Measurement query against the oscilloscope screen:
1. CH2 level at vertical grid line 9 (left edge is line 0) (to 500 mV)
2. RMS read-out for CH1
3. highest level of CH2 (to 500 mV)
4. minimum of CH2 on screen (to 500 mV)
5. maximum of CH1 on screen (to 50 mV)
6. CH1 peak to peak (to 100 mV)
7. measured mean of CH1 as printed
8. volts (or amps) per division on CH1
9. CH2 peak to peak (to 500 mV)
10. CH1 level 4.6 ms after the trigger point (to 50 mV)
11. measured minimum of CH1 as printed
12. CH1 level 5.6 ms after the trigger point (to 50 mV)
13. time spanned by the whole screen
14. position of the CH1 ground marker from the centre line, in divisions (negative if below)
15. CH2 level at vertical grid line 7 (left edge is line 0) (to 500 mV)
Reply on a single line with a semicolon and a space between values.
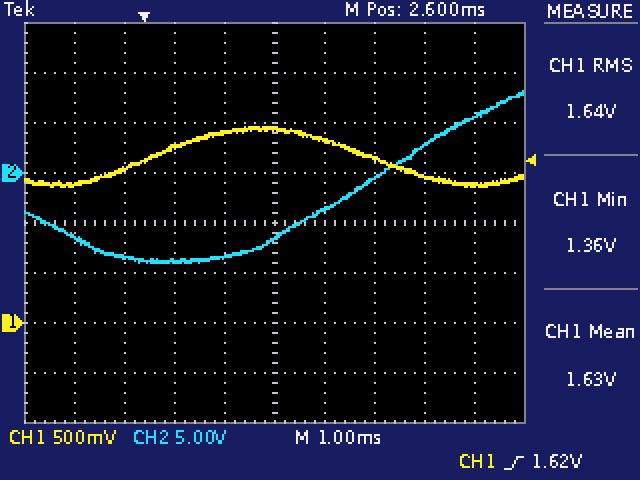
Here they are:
5.5 V; 1.64 V; 8.0 V; -9.0 V; 1.95 V; 600 mV; 1.63 V; 500 mV; 17.0 V; 1.65 V; 1.36 V; 1.45 V; 10 ms; -2.0 div; -500 mV
